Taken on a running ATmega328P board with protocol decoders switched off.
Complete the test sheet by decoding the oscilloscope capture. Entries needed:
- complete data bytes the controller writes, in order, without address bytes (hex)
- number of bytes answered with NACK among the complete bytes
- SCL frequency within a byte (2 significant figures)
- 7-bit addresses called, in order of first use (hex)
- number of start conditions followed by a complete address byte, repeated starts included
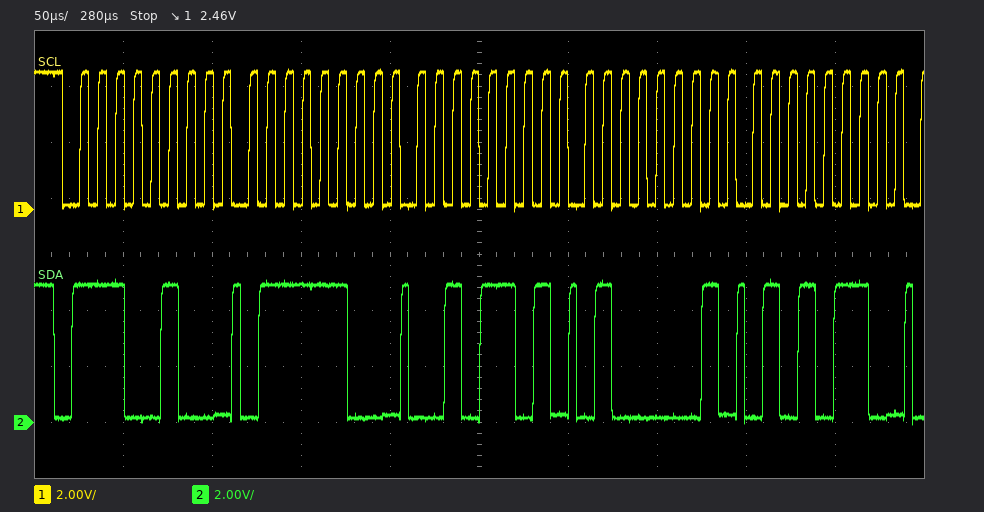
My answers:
7C 2D 41 56
0
100 kHz
0x72
1
